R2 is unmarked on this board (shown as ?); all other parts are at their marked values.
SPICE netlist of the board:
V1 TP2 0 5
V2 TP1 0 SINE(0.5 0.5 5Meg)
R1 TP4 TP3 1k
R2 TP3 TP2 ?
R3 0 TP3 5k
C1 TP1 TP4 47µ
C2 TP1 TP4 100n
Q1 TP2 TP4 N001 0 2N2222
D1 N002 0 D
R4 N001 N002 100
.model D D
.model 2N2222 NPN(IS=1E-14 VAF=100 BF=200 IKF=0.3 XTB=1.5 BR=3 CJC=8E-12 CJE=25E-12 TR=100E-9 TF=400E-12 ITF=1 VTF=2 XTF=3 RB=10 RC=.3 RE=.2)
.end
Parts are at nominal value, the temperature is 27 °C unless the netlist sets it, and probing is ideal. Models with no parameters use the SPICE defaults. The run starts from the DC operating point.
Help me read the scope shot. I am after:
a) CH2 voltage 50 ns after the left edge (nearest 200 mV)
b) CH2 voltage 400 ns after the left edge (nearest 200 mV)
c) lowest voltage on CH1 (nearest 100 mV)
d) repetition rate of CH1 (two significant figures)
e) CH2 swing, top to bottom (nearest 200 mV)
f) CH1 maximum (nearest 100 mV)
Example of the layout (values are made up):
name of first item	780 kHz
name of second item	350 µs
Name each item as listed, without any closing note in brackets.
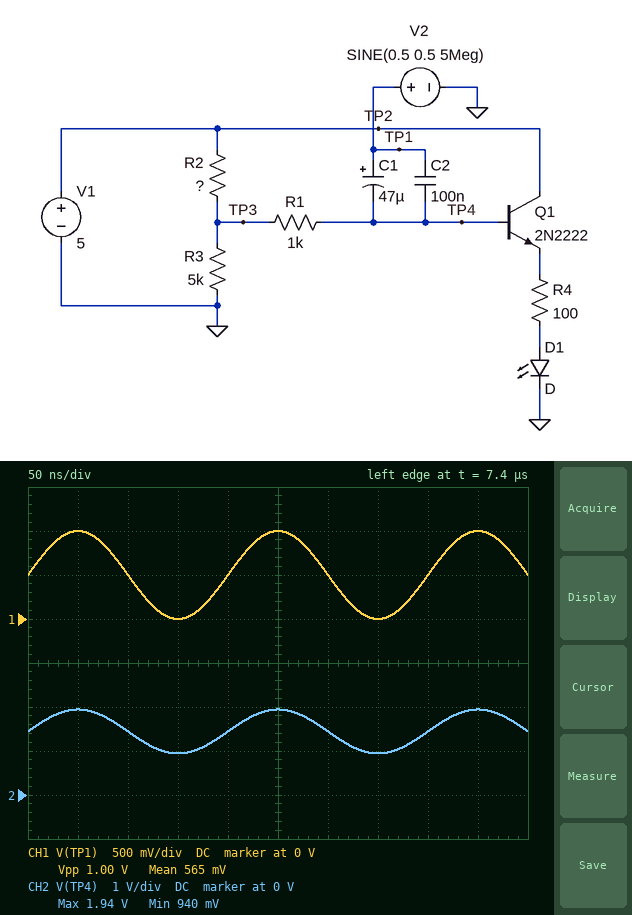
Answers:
CH2 voltage 50 ns after the left edge	2.0 V
CH2 voltage 400 ns after the left edge	1.4 V
lowest voltage on CH1	0 V
repetition rate of CH1	5.0 MHz
CH2 swing, top to bottom	1.0 V
CH1 maximum	1.0 V
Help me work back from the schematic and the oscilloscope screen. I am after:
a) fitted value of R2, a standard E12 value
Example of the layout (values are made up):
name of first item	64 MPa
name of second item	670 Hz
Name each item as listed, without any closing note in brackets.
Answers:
fitted value of R2, a standard E12 value	12 kΩ
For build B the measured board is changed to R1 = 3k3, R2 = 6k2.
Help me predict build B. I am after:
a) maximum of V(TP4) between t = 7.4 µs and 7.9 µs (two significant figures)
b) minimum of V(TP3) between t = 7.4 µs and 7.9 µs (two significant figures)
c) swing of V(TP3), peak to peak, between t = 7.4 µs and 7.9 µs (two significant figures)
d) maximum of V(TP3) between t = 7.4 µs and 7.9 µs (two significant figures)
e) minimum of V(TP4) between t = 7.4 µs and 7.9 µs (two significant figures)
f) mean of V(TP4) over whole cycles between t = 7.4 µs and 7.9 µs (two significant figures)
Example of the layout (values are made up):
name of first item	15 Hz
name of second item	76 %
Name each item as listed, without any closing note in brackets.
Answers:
maximum of V(TP4) between t = 7.4 µs and 7.9 µs	2.5 V
minimum of V(TP3) between t = 7.4 µs and 7.9 µs	1.9 V
swing of V(TP3), peak to peak, between t = 7.4 µs and 7.9 µs	460 mV
maximum of V(TP3) between t = 7.4 µs and 7.9 µs	2.4 V
minimum of V(TP4) between t = 7.4 µs and 7.9 µs	1.5 V
mean of V(TP4) over whole cycles between t = 7.4 µs and 7.9 µs	2.0 V
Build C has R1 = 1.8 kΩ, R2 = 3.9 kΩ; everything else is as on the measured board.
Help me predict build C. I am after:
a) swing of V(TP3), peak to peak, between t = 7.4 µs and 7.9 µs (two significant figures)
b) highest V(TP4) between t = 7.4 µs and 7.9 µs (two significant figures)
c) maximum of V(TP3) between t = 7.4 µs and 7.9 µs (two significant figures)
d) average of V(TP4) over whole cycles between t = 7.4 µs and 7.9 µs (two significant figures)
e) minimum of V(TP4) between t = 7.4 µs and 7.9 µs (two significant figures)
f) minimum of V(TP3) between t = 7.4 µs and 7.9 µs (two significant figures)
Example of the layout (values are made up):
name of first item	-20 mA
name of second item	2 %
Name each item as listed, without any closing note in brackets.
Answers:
swing of V(TP3), peak to peak, between t = 7.4 µs and 7.9 µs	550 mV
highest V(TP4) between t = 7.4 µs and 7.9 µs	3.1 V
maximum of V(TP3) between t = 7.4 µs and 7.9 µs	3.0 V
average of V(TP4) over whole cycles between t = 7.4 µs and 7.9 µs	2.6 V
minimum of V(TP4) between t = 7.4 µs and 7.9 µs	2.1 V
minimum of V(TP3) between t = 7.4 µs and 7.9 µs	2.4 V
